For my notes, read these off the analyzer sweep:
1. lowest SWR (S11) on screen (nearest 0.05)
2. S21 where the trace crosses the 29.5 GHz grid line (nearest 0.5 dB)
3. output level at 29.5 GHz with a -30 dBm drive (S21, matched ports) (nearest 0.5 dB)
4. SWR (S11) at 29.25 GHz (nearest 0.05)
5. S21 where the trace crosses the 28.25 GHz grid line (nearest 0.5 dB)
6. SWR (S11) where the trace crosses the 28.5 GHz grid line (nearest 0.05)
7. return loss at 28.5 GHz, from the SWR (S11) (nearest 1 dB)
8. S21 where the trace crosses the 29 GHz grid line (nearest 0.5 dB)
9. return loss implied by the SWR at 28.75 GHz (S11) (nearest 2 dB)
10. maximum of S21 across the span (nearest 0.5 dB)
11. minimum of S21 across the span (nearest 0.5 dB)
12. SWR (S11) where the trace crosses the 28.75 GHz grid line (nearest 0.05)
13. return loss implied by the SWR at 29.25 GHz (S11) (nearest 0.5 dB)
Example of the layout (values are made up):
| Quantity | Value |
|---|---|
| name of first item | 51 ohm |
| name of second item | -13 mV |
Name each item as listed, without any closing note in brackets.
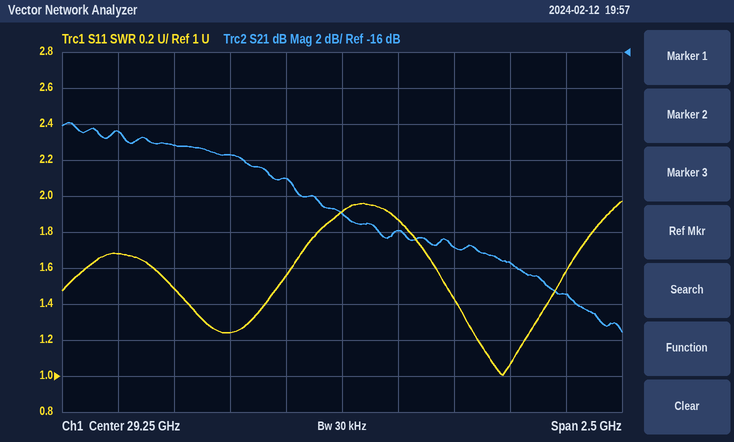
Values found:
| Quantity | Value |
|---|---|
| lowest SWR (S11) on screen | 1.00 |
| S21 where the trace crosses the 29.5 GHz grid line | -26.0 dB |
| output level at 29.5 GHz with a -30 dBm drive (S21, matched ports) | -56.0 dBm |
| SWR (S11) at 29.25 GHz | 1.90 |
| S21 where the trace crosses the 28.25 GHz grid line | -20.5 dB |
| SWR (S11) where the trace crosses the 28.5 GHz grid line | 1.50 |
| return loss at 28.5 GHz, from the SWR (S11) | 14 dB |
| S21 where the trace crosses the 29 GHz grid line | -23.0 dB |
| return loss implied by the SWR at 28.75 GHz (S11) | 20 dB |
| maximum of S21 across the span | -20.0 dB |
| minimum of S21 across the span | -31.5 dB |
| SWR (S11) where the trace crosses the 28.75 GHz grid line | 1.25 |
| return loss implied by the SWR at 29.25 GHz (S11) | 10.0 dB |
